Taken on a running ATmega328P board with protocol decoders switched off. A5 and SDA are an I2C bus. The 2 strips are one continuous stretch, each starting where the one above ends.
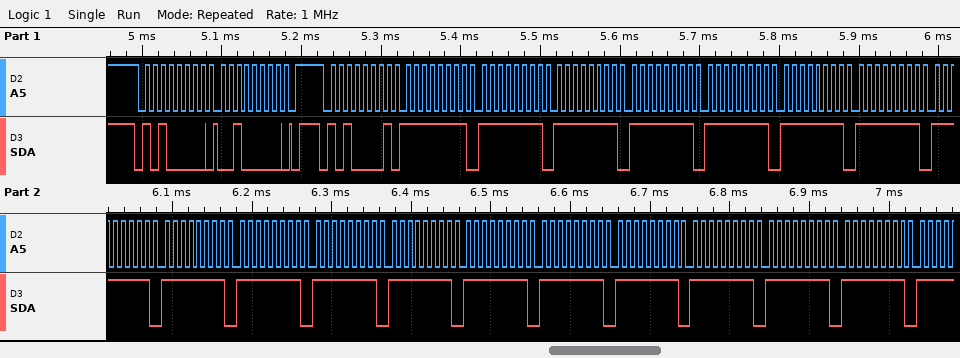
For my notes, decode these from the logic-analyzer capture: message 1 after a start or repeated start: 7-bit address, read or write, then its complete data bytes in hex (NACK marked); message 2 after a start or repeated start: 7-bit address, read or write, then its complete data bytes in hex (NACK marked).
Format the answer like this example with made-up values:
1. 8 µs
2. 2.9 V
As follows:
1. 0x50 write: 20
2. 0x50 read: FF FF FF FF FF FF FF FF FF FF FF FF FF FF FF FF FF FF
